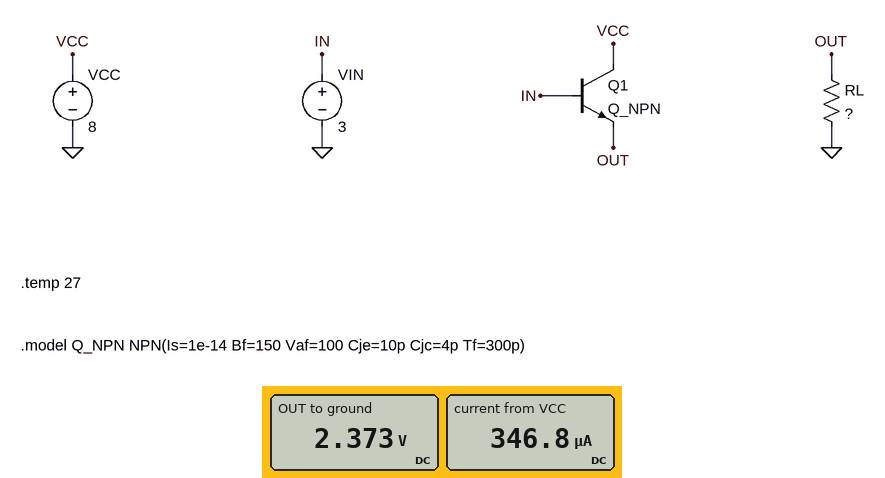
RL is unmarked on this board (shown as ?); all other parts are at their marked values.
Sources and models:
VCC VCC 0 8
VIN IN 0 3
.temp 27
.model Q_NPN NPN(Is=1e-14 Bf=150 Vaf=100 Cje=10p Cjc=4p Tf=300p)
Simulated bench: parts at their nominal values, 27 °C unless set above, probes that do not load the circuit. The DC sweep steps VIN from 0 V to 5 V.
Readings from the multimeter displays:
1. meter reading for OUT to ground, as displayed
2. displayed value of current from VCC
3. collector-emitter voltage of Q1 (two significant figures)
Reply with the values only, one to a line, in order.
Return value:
2.373 V
346.8 µA
5.6 V
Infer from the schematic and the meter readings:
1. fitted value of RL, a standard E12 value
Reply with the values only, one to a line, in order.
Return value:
6.8 kΩ
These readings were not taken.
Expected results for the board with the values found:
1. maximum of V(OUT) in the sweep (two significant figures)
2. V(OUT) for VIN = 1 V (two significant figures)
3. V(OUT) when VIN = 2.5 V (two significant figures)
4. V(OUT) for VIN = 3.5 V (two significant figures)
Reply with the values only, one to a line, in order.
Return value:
4.4 V
420 mV
1.9 V
2.9 V
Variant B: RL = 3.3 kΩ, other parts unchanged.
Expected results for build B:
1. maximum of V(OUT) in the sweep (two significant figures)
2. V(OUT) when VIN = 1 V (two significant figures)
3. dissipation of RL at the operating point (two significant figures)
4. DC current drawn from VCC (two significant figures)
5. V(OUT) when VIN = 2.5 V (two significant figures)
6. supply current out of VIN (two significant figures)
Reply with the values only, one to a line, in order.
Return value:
4.3 V
400 mV
1.7 mW
710 µA
1.9 V
4.5 µA
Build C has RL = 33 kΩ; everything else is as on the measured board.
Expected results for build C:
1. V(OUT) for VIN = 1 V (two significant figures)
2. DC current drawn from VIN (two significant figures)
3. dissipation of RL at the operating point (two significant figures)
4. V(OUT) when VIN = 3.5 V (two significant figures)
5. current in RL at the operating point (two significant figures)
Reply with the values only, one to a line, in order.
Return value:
460 mV
460 nA
180 µW
2.9 V
73 µA
